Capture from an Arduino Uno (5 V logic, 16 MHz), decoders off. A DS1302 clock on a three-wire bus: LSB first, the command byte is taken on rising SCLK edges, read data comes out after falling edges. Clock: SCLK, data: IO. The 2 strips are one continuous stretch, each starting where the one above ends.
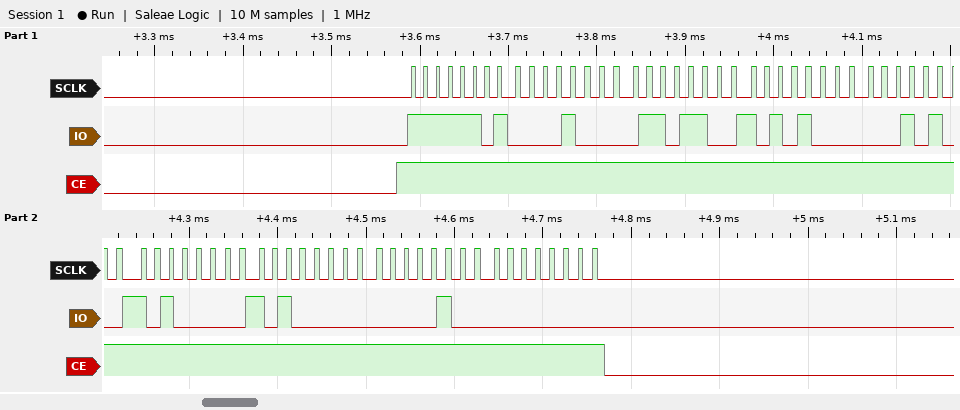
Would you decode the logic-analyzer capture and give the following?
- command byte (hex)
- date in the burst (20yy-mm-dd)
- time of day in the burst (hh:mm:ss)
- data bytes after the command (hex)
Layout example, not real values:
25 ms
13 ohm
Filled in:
0xBF
2020-05-28
15:36:10
10 36 15 28 05 05 20 00
